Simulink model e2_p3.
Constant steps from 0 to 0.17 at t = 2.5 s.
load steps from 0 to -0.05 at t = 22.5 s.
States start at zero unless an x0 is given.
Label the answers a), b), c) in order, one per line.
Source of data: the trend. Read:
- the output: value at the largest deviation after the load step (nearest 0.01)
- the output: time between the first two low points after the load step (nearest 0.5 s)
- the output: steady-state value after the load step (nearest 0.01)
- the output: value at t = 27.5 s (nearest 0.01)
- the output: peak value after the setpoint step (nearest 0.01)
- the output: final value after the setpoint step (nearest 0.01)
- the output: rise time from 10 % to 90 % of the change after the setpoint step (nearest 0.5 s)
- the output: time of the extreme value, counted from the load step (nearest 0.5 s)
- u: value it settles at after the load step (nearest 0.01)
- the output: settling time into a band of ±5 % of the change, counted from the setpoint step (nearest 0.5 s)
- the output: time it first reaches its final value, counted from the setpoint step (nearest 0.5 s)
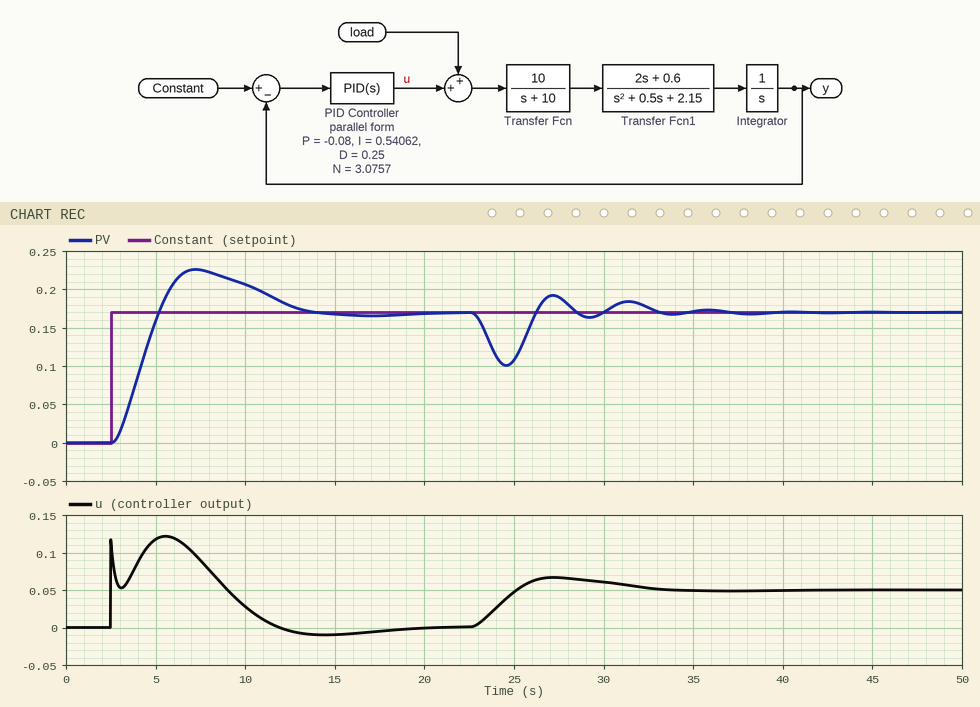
a) 0.10
b) 4.5 s
c) 0.17
d) 0.19
e) 0.23
f) 0.17
g) 2.0 s
h) 2.0 s
i) 0.05
j) 10.0 s
k) 2.5 s
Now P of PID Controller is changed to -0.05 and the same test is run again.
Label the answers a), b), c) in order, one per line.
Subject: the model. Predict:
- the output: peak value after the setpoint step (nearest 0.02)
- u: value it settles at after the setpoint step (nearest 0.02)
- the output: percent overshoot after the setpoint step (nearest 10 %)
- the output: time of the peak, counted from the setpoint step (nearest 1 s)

a) 0.22
b) 0.00
c) 30 %
d) 5 s
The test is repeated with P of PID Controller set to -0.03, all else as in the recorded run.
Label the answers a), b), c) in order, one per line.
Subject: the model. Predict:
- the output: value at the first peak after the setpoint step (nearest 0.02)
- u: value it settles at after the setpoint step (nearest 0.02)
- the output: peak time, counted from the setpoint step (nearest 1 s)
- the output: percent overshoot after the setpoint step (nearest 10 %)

a) 0.22
b) 0.00
c) 6 s
d) 30 %
